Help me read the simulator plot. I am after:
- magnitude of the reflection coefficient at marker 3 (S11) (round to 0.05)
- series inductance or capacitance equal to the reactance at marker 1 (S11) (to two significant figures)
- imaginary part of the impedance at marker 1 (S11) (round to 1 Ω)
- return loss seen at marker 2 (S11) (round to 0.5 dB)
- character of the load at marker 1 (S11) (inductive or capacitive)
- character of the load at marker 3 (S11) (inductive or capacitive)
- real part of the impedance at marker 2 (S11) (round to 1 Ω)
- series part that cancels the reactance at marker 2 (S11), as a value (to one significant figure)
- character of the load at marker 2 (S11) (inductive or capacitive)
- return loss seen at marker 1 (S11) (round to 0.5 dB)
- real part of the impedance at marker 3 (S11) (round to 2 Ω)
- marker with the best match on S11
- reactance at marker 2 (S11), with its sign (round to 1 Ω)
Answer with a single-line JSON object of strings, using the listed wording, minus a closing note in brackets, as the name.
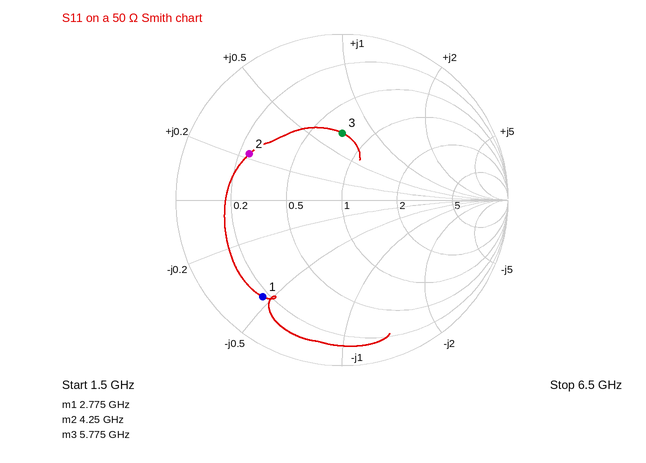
{"magnitude of the reflection coefficient at marker 3 (S11)": "0.40", "series inductance or capacitance equal to the reactance at marker 1 (S11)": "2.5 pF", "imaginary part of the impedance at marker 1 (S11)": "-23 Ω", "return loss seen at marker 2 (S11)": "4.0 dB", "character of the load at marker 1 (S11)": "capacitive", "character of the load at marker 3 (S11)": "inductive", "real part of the impedance at marker 2 (S11)": "12 Ω", "series part that cancels the reactance at marker 2 (S11), as a value": "3 pF", "character of the load at marker 2 (S11)": "inductive", "return loss seen at marker 1 (S11)": "2.5 dB", "real part of the impedance at marker 3 (S11)": "36 Ω", "marker with the best match on S11": "marker 3", "reactance at marker 2 (S11), with its sign": "+11 Ω"}
